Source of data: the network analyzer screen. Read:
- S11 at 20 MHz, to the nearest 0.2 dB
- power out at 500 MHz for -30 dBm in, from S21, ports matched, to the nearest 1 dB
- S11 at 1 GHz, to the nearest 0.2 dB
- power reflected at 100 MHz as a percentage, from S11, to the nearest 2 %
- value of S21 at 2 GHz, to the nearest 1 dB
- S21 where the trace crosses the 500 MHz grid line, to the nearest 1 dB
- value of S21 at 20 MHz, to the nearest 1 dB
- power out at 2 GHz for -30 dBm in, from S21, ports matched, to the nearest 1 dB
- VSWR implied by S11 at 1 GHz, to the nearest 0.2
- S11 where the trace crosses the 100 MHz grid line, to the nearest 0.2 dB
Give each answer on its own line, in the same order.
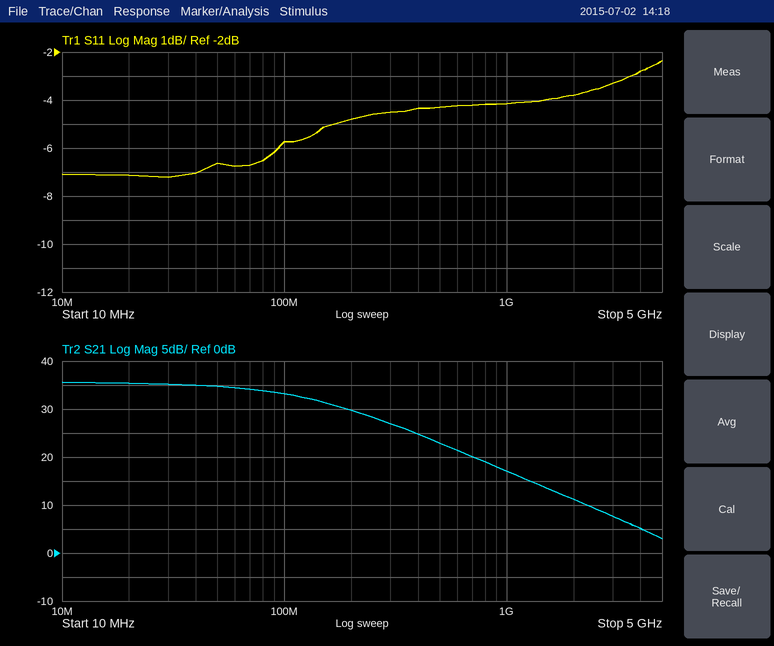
-7.2 dB
-7 dBm
-4.2 dB
26 %
11 dB
23 dB
35 dB
-19 dBm
4.2
-5.8 dB
